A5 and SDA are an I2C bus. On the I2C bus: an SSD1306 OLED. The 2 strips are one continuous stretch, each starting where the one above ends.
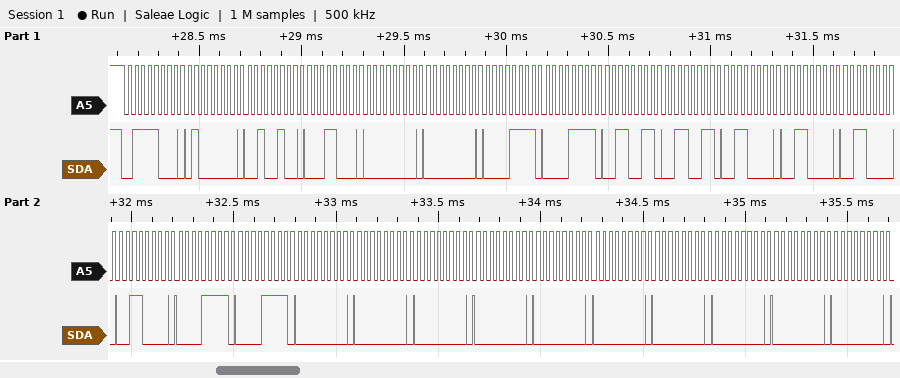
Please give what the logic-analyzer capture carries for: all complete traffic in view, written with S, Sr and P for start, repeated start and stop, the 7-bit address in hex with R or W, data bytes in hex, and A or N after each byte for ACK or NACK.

S 3CW A 40 A 24 A 18 A 00 A 00 A 0F A 0F A 33 A 33 A 30 A 30 A 30 A 30 A 0F A 0F A 00 A 00 A 00 A 00 A 00 A 00 A 00 A 00 A 00 A 00 A
